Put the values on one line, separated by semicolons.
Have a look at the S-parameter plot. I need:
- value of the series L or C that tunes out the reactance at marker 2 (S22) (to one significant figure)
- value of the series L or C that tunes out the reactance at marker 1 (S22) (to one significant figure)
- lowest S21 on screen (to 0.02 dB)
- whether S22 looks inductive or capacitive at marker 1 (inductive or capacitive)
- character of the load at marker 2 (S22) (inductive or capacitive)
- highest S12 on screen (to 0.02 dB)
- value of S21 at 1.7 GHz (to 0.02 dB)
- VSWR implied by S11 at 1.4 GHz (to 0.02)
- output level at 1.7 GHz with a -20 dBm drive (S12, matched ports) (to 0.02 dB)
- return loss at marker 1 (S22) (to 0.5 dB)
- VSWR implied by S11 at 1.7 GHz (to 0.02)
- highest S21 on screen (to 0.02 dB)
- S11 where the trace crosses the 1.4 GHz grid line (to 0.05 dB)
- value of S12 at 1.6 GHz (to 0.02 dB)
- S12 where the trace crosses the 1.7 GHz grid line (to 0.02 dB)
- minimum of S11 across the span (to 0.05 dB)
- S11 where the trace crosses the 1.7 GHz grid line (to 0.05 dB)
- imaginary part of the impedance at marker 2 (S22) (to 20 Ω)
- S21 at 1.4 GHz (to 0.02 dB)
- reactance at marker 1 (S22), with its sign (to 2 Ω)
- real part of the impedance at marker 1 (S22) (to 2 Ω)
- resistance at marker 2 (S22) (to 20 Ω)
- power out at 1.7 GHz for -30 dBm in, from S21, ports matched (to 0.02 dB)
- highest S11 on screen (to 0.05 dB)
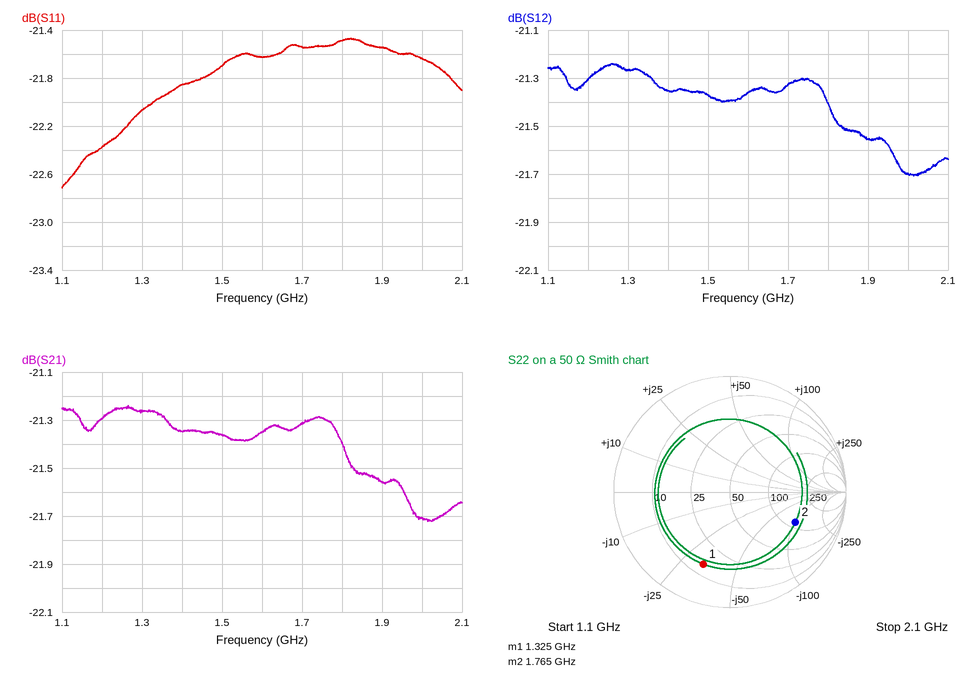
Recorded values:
9 nH; 4 nH; -21.72 dB; capacitive; capacitive; -21.24 dB; -21.32 dB; 1.18; -41.32 dBm; 3.5 dB; 1.18; -21.24 dB; -21.85 dB; -21.36 dB; -21.32 dB; -22.70 dB; -21.55 dB; -100 Ω; -21.34 dB; -32 Ω; 14 Ω; 120 Ω; -51.32 dBm; -21.45 dB
